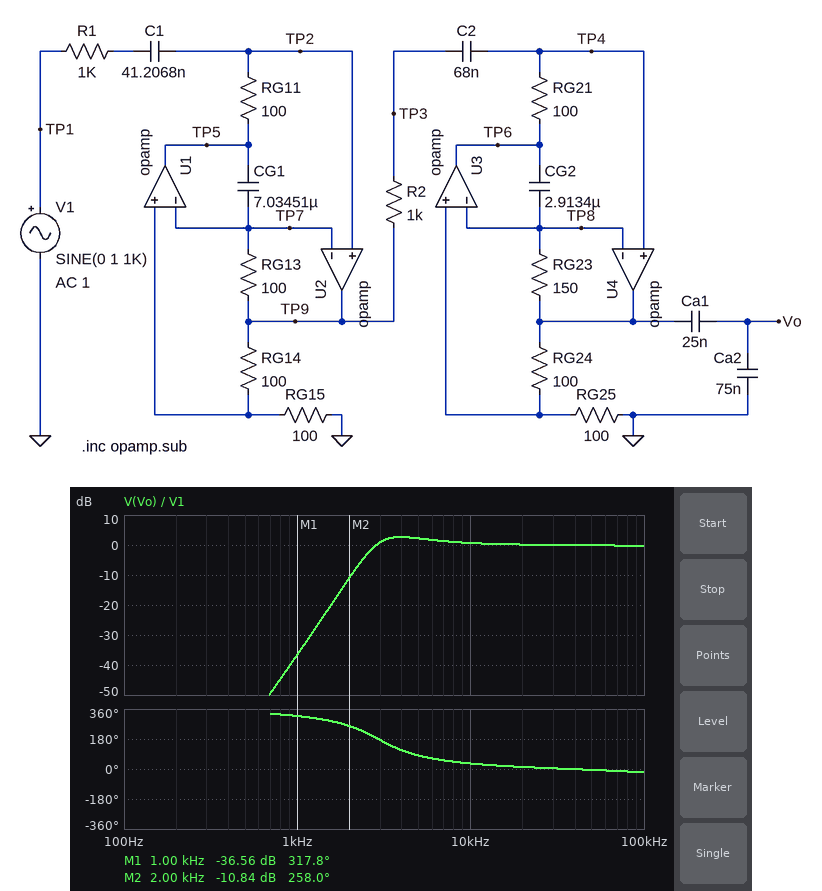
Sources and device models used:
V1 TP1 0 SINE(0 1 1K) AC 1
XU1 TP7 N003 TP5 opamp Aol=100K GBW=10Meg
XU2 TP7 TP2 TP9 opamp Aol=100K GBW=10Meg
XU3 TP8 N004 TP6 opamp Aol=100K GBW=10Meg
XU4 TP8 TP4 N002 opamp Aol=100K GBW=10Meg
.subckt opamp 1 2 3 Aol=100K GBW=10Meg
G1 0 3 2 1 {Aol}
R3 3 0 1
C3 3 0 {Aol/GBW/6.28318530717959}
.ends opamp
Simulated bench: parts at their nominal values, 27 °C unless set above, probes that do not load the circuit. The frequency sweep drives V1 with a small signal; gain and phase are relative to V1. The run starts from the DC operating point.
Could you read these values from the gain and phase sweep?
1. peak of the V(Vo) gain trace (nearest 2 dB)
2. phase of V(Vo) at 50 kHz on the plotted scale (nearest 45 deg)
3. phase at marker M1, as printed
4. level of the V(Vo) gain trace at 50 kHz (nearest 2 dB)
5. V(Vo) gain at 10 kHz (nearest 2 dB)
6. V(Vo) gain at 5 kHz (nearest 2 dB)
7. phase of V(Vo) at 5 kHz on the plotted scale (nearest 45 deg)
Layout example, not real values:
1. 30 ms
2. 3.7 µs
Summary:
1. 2 dB
2. 0 deg
3. 317.8 deg
4. 0 dB
5. 0 dB
6. 2 dB
7. 90 deg
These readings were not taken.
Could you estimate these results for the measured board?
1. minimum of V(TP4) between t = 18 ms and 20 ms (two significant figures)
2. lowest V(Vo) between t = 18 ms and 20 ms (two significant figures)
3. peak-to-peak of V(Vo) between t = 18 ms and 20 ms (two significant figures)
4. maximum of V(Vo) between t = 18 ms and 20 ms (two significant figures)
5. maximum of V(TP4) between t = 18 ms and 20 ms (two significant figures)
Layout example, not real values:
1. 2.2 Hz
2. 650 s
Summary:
1. -30 mV
2. -15 mV
3. 30 mV
4. 15 mV
5. 30 mV
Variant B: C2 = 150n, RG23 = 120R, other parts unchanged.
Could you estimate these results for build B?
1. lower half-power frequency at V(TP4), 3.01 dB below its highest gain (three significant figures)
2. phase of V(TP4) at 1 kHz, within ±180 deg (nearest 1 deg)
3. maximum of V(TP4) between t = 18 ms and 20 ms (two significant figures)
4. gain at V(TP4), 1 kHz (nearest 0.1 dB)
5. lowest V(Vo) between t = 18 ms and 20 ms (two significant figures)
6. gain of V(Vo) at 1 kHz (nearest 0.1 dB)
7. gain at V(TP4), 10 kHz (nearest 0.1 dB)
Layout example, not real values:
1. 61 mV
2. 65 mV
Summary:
1. 2.80 kHz
2. -66 deg
3. 42 mV
4. -27.6 dB
5. -21 mV
6. -33.6 dB
7. 6.1 dB
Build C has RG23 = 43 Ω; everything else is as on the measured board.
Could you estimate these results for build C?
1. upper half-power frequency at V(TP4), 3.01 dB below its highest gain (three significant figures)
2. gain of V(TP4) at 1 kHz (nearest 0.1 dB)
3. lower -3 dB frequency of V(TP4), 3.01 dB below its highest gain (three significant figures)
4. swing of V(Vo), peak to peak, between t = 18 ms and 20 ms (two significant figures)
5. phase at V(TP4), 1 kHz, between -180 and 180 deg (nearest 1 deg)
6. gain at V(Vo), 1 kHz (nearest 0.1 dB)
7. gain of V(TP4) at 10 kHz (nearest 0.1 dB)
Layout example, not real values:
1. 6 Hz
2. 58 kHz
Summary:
1. 319 kHz
2. -42.0 dB
3. 8.94 kHz
4. 7.9 mV
5. -40 deg
6. -48.1 dB
7. 3.4 dB
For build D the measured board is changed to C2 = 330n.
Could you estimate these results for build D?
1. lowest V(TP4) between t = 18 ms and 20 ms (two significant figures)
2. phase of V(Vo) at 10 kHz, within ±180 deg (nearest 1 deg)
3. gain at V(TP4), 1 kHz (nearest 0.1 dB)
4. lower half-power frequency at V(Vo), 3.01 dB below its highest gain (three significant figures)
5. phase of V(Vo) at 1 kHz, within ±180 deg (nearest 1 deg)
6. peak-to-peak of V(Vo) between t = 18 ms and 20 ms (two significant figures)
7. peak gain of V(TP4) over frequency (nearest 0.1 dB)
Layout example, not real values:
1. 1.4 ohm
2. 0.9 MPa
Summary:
1. -67 mV
2. 32 deg
3. -23.5 dB
4. 2.72 kHz
5. -95 deg
6. 67 mV
7. 6.8 dB
